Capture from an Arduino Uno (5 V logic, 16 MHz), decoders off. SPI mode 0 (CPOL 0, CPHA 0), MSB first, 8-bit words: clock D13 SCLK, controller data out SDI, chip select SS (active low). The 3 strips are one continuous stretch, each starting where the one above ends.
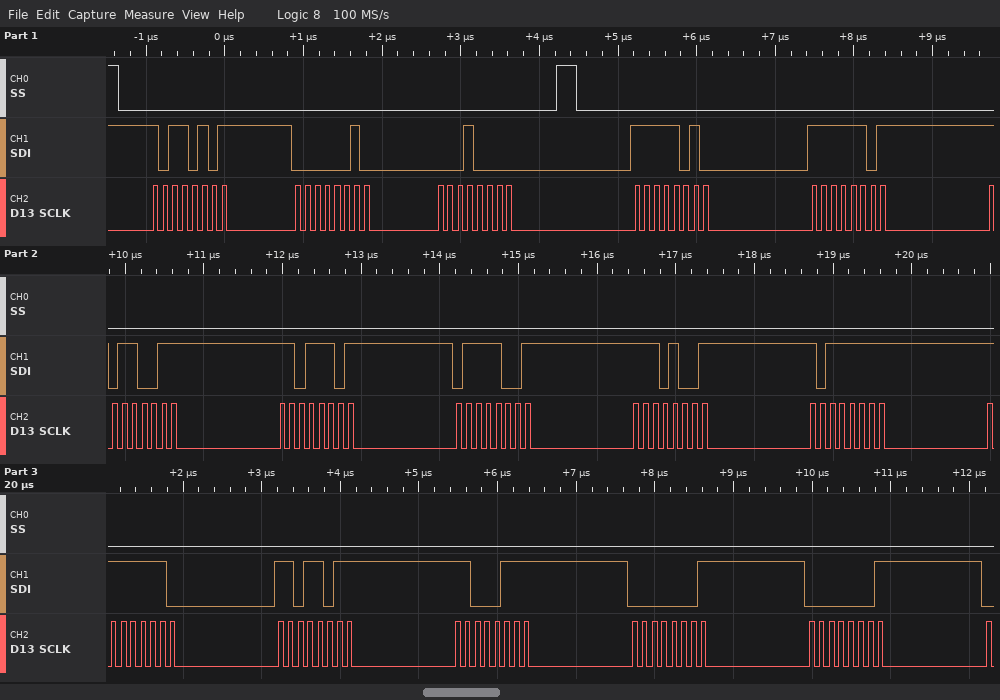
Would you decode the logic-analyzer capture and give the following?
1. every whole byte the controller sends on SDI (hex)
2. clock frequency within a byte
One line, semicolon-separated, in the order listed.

0xB5 0x02 0x10 0xFA 0xFD 0xB3 0xDD 0x79 0xE9 0xBF 0xFE 0xDB 0xC7 0x01 0x01; 8 MHz
